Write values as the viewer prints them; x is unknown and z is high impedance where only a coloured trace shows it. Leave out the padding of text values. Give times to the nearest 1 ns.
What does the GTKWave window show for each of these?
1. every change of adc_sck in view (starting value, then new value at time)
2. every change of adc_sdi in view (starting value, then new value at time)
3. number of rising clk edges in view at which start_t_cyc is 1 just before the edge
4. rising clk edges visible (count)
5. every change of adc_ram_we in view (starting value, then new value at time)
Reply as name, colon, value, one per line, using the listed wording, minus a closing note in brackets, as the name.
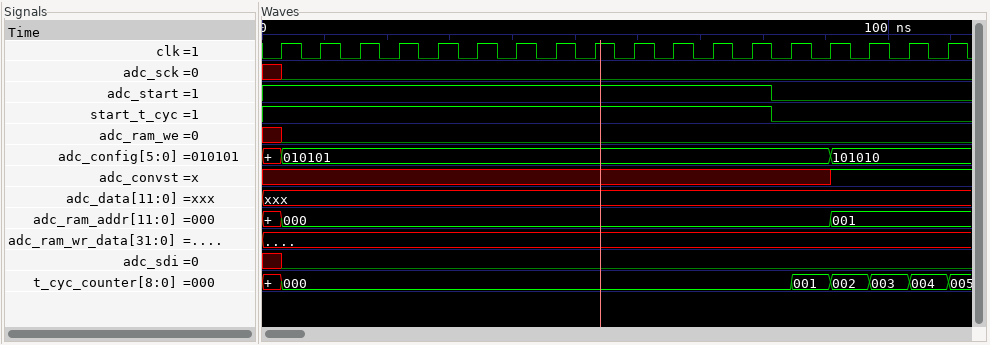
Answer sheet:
every change of adc_sck in view: x, 0 at 3 ns
every change of adc_sdi in view: x, 0 at 3 ns
number of rising clk edges in view at which start_t_cyc is 1 just before the edge: 13
rising clk edges visible: 18
every change of adc_ram_we in view: x, 0 at 3 ns
